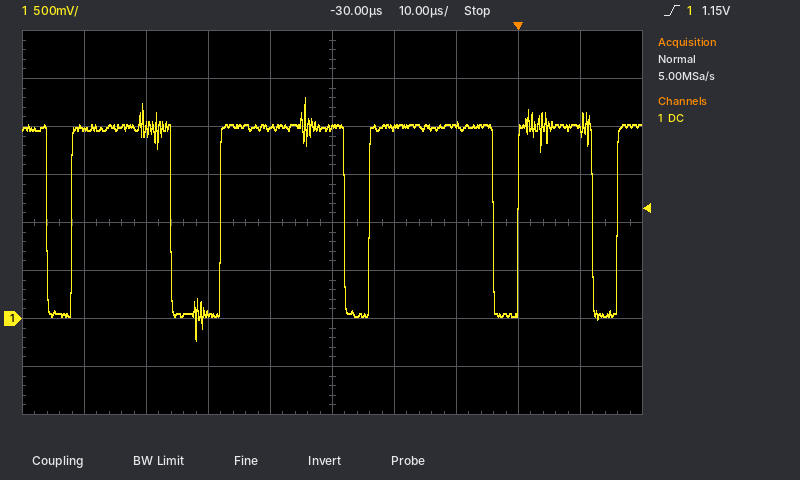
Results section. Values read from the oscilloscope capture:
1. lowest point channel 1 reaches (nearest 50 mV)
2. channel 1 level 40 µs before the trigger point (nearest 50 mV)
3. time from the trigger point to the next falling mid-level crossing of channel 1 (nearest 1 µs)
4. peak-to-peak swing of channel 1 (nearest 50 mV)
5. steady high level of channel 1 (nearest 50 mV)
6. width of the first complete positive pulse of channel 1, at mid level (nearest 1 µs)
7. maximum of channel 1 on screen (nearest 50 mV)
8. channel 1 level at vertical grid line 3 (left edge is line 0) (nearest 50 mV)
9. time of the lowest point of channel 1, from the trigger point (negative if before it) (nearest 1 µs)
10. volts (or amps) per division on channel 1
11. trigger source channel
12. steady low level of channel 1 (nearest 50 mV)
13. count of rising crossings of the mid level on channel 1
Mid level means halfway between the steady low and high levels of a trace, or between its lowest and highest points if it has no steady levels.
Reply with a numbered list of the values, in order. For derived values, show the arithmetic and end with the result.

1. -250 mV
2. 2.00 V
3. 12 µs
4. 2.30 V − (-250 mV) = 2.55 V
5. 2.00 V
6. 16 µs
7. 2.30 V
8. 50 mV
9. -52 µs
10. 500 mV
11. channel 1
12. 50 mV
13. 5
